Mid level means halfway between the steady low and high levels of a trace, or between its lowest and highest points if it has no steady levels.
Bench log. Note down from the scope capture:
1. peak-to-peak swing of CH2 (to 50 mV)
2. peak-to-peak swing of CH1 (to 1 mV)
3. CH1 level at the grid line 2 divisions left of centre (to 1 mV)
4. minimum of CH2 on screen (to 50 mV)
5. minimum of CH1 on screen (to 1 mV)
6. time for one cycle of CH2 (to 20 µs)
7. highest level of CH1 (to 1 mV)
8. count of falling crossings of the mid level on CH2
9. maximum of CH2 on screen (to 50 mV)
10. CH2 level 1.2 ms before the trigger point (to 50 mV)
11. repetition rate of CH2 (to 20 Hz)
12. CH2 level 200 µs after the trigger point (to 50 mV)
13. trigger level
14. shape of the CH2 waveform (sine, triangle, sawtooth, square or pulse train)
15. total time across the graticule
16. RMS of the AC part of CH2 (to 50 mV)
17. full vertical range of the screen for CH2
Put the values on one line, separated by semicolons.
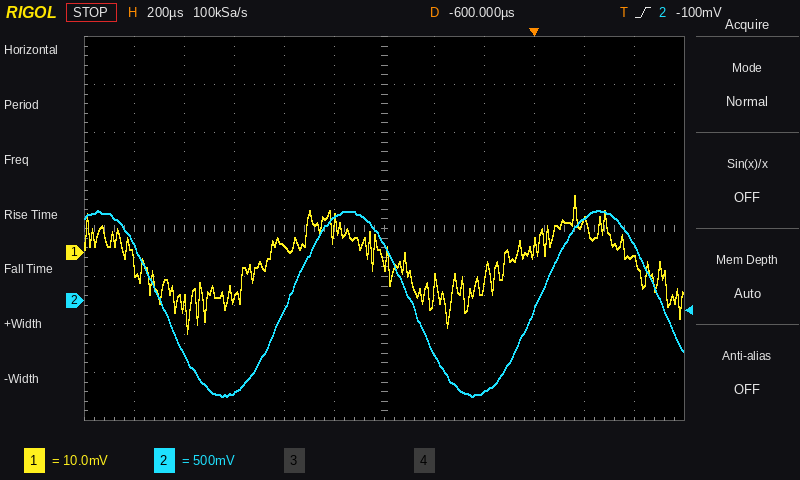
1.95 V; 29 mV; 1 mV; -1.00 V; -17 mV; 1.00 ms; 12 mV; 3; 950 mV; -950 mV; 1.00 kHz; 850 mV; -100 mV; sine; 2.4 ms; 700 mV; 4 V
